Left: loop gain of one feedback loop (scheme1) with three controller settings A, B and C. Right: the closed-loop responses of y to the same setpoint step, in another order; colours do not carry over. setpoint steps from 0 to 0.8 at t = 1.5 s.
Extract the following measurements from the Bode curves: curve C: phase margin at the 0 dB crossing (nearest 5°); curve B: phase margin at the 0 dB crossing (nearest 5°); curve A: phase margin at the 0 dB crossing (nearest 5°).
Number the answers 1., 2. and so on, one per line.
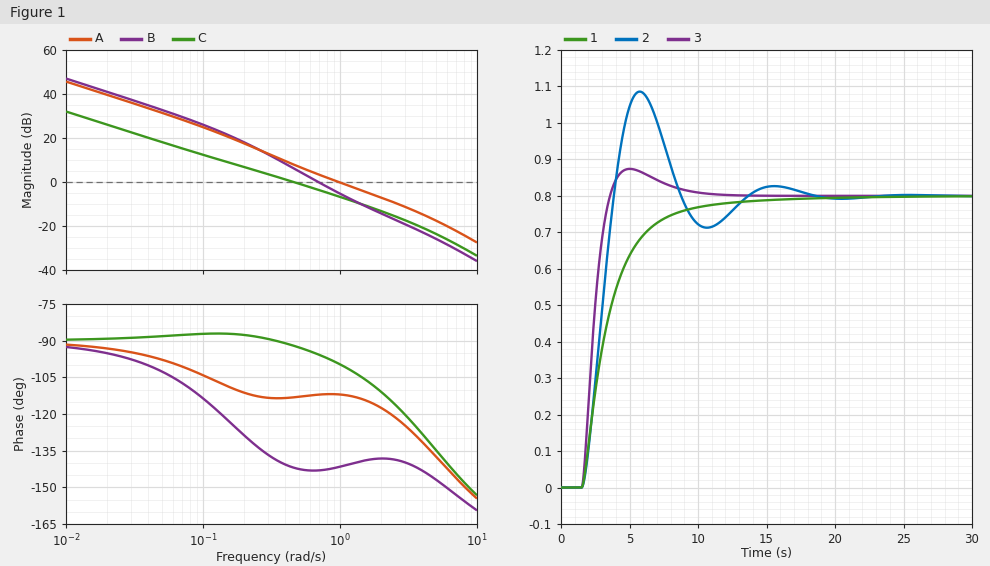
1. 90°
2. 35°
3. 70°
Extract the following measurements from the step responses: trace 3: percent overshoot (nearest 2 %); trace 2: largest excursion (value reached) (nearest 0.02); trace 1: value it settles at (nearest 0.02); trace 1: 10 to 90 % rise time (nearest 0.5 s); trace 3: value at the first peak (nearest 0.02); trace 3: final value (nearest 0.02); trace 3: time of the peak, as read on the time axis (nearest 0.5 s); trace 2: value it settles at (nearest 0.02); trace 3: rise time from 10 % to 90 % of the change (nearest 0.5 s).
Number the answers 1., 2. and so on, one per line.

1. 10 %
2. 1.08
3. 0.80
4. 5.0 s
5. 0.88
6. 0.80
7. 5.0 s
8. 0.80
9. 1.5 s
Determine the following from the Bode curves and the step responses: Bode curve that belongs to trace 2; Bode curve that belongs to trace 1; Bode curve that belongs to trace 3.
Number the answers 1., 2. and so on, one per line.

1. B
2. C
3. A
